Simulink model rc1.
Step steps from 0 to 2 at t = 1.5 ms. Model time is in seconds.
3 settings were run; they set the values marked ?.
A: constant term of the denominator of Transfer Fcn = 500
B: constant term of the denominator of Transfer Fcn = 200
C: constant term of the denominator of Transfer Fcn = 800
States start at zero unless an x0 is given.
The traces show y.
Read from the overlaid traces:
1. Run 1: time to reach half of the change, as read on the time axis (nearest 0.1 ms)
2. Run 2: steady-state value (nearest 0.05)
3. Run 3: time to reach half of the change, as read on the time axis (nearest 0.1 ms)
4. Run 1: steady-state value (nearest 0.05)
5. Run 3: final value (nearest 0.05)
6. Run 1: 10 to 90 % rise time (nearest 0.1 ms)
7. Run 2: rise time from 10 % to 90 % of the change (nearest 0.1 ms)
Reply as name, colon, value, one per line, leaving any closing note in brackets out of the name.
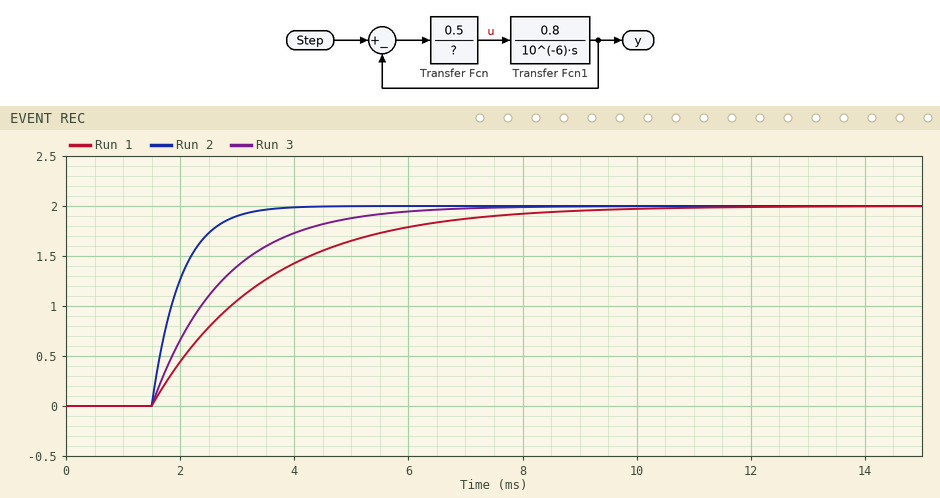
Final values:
Run 1: time to reach half of the change, as read on the time axis: 2.9 ms
Run 2: steady-state value: 2.00
Run 3: time to reach half of the change, as read on the time axis: 2.4 ms
Run 1: steady-state value: 2.00
Run 3: final value: 2.00
Run 1: 10 to 90 % rise time: 4.4 ms
Run 2: rise time from 10 % to 90 % of the change: 1.1 ms
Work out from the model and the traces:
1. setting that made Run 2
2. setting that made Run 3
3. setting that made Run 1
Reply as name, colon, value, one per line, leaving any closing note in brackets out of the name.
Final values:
setting that made Run 2: B
setting that made Run 3: A
setting that made Run 1: C
